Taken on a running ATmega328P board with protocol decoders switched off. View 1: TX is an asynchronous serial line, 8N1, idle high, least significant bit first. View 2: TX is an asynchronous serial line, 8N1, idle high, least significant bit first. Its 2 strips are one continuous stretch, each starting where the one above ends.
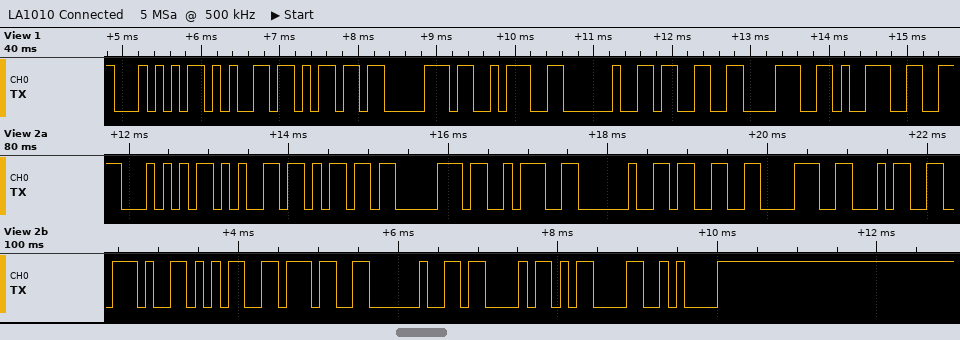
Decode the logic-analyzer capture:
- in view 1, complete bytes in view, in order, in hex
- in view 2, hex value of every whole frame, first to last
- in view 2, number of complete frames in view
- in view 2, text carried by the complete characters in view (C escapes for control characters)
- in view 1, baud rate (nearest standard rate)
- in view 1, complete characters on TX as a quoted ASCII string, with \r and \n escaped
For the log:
54 65 6D 70 3A 20 33 38 39
54 65 6D 70 3A 20 33 38 34 2E 35 37 20 43 0D 0A
16
"Temp: 384.57 C\r\n"
9600 baud
"Temp: 389"
